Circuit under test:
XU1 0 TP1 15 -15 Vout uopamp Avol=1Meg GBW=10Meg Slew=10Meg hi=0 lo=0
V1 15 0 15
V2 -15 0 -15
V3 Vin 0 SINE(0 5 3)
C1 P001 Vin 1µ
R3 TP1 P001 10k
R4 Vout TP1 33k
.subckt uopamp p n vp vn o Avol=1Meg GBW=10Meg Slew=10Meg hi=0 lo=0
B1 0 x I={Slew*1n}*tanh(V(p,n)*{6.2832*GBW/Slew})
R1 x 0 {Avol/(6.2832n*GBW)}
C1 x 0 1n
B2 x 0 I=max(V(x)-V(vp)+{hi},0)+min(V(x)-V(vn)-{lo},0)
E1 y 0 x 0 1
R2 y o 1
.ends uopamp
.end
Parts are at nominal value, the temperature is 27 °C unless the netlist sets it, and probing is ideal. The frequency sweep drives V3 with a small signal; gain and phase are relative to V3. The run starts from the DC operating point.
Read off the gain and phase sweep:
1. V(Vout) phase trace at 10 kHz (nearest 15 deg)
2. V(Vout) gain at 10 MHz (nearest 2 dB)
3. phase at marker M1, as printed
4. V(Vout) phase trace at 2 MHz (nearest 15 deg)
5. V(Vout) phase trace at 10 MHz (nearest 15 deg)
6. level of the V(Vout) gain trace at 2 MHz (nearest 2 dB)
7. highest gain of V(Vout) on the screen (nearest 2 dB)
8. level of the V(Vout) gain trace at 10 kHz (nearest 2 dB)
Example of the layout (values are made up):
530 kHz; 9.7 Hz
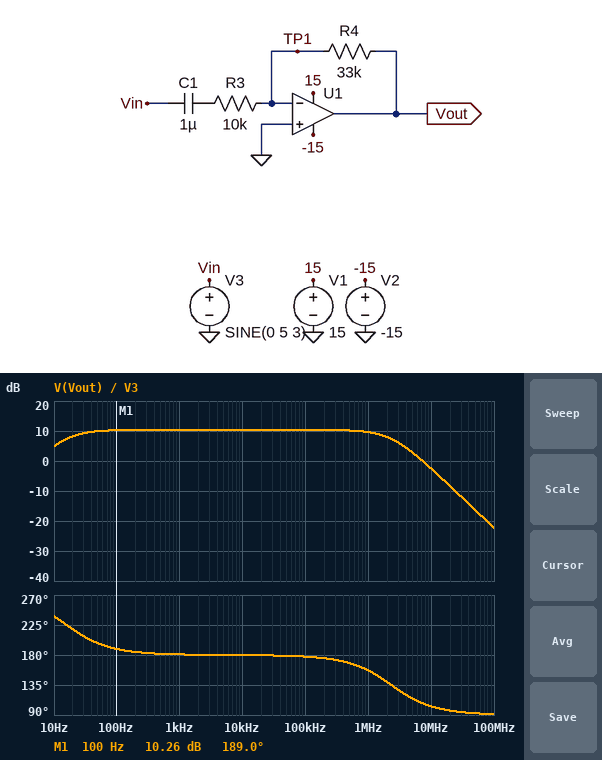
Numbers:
180 deg; -2 dB; 189.0 deg; 135 deg; 105 deg; 8 dB; 10 dB; 10 dB
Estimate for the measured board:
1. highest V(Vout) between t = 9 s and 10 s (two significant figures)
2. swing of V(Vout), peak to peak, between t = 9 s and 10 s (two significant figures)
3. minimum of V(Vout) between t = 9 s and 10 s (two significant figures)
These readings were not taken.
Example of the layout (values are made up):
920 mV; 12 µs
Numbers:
3.1 V; 6.1 V; -3.1 V
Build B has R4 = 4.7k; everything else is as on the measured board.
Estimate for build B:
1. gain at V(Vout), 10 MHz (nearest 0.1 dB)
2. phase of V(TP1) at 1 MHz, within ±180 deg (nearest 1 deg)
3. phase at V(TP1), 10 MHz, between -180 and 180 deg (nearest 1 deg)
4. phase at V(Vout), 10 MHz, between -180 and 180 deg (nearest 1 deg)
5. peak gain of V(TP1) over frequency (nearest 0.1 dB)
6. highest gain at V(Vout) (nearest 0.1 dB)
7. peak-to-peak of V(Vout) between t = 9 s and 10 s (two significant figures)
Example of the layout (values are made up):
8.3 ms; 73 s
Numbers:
-11.6 dB; 82 deg; 34 deg; 124 deg; -9.9 dB; -6.6 dB; 870 mV
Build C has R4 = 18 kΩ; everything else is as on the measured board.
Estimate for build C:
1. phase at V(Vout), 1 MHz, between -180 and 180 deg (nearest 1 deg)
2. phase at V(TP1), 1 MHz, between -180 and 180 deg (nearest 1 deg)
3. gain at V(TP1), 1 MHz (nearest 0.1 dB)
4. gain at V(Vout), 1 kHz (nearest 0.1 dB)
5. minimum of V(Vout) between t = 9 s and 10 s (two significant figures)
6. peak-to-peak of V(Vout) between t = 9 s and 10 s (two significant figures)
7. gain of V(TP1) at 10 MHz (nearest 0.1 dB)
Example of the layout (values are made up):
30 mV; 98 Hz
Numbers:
164 deg; 74 deg; -15.2 dB; 5.1 dB; -1.7 V; 3.3 V; -4.4 dB
